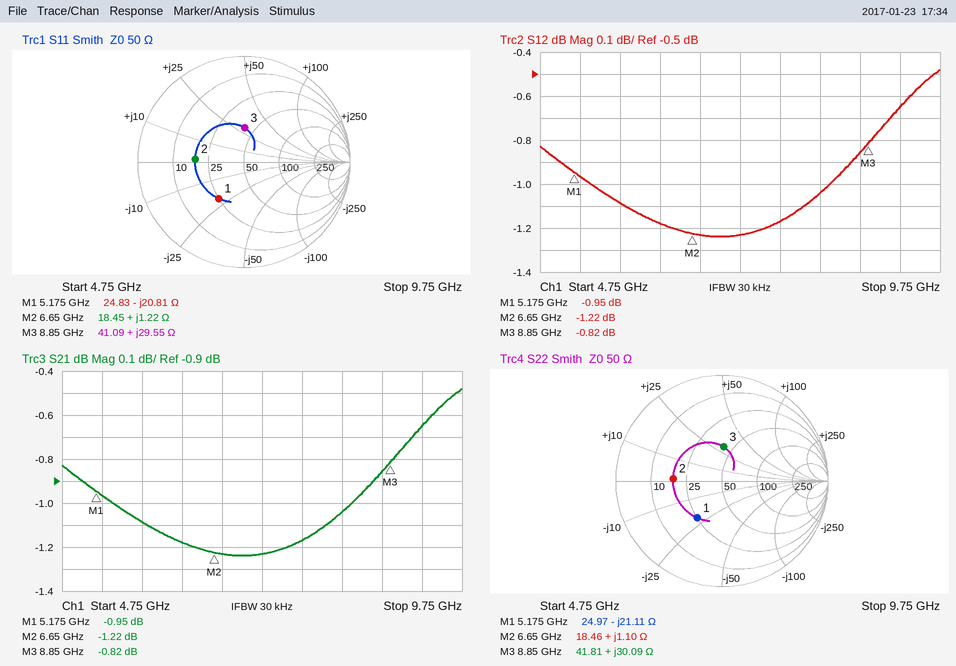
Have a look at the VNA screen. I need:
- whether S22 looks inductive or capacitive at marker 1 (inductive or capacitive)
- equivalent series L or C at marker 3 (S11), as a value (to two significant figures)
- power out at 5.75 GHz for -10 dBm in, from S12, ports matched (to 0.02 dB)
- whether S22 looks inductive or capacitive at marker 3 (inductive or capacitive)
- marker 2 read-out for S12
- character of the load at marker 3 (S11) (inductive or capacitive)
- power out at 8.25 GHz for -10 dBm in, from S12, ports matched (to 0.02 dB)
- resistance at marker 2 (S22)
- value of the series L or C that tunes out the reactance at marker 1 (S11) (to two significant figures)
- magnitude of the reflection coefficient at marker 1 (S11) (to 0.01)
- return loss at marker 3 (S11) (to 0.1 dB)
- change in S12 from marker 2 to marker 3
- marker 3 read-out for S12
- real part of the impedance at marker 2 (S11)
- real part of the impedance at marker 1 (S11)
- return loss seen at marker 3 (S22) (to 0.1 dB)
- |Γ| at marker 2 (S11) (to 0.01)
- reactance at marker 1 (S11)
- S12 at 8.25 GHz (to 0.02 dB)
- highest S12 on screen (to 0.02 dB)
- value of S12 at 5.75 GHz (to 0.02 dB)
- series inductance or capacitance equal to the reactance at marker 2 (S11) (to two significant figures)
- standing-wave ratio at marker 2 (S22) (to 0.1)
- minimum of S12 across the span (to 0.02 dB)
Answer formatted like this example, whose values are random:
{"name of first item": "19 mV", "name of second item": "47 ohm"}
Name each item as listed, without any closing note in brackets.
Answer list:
{"whether S22 looks inductive or capacitive at marker 1": "capacitive", "equivalent series L or C at marker 3 (S11), as a value": "530 pH", "power out at 5.75 GHz for -10 dBm in, from S12, ports matched": "-11.08 dBm", "whether S22 looks inductive or capacitive at marker 3": "inductive", "marker 2 read-out for S12": "-1.22 dB", "character of the load at marker 3 (S11)": "inductive", "power out at 8.25 GHz for -10 dBm in, from S12, ports matched": "-11.04 dBm", "resistance at marker 2": "18.46 Ω", "value of the series L or C that tunes out the reactance at marker 1 (S11)": "640 pH", "magnitude of the reflection coefficient at marker 1 (S11)": "0.42", "return loss at marker 3 (S11)": "9.8 dB", "change in S12 from marker 2 to marker 3": "0.40 dB", "marker 3 read-out for S12": "-0.82 dB", "real part of the impedance at marker 2": "18.45 Ω", "real part of the impedance at marker 1": "24.83 Ω", "return loss seen at marker 3 (S22)": "9.8 dB", "|Γ| at marker 2 (S11)": "0.46", "reactance at marker 1": "-20.81 Ω", "S12 at 8.25 GHz": "-1.04 dB", "highest S12 on screen": "-0.48 dB", "value of S12 at 5.75 GHz": "-1.08 dB", "series inductance or capacitance equal to the reactance at marker 2 (S11)": "29 pH", "standing-wave ratio at marker 2 (S22)": "2.7", "minimum of S12 across the span": "-1.24 dB"}
